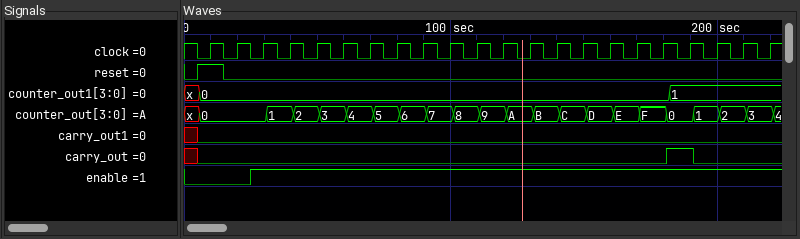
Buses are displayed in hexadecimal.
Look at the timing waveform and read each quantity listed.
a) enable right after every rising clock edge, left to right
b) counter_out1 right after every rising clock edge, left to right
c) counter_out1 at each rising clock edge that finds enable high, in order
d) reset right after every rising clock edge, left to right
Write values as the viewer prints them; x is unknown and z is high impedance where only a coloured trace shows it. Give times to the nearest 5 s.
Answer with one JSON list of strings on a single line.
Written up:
["0 0 1 1 1 1 1 1 1 1 1 1 1 1 1 1 1 1 1 1 1 1", "0, 0, 0, 0, 0, 0, 0, 0, 0, 0, 0, 0, 0, 0, 0, 0, 0, 0, 1, 1, 1, 1", "0, 0, 0, 0, 0, 0, 0, 0, 0, 0, 0, 0, 0, 0, 0, 0, 1, 1, 1, 1", "1 0 0 0 0 0 0 0 0 0 0 0 0 0 0 0 0 0 0 0 0 0"]
